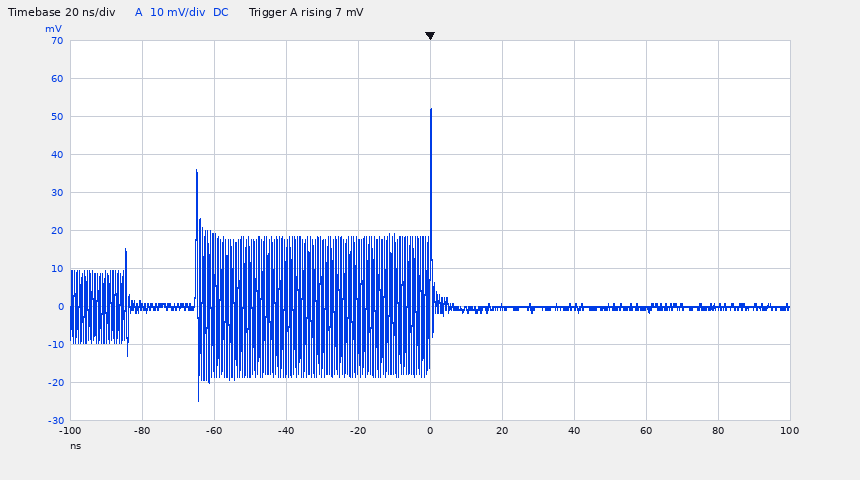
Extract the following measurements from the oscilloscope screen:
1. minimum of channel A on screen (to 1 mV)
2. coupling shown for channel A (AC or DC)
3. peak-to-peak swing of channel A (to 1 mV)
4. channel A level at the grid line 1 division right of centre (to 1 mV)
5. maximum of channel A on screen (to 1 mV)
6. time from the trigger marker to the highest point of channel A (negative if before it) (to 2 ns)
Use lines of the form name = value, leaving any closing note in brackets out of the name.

minimum of channel A on screen = -25 mV
coupling shown for channel A = DC
peak-to-peak swing of channel A = 77 mV
channel A level at the grid line 1 division right of centre = 0 mV
maximum of channel A on screen = 52 mV
time from the trigger marker to the highest point of channel A (negative if before it) = 0 ns
